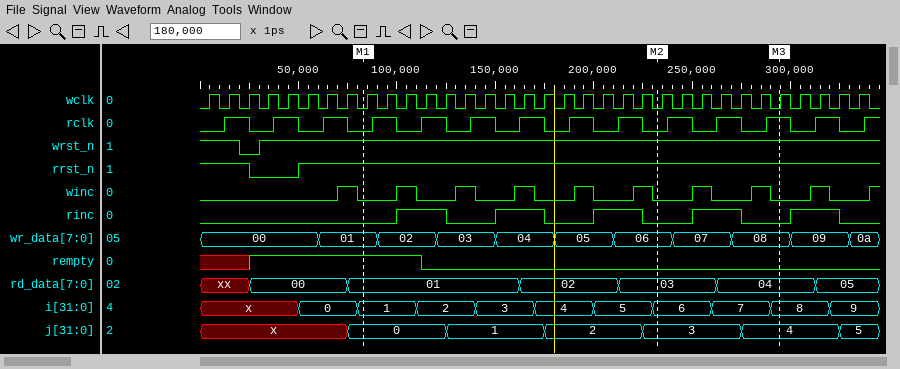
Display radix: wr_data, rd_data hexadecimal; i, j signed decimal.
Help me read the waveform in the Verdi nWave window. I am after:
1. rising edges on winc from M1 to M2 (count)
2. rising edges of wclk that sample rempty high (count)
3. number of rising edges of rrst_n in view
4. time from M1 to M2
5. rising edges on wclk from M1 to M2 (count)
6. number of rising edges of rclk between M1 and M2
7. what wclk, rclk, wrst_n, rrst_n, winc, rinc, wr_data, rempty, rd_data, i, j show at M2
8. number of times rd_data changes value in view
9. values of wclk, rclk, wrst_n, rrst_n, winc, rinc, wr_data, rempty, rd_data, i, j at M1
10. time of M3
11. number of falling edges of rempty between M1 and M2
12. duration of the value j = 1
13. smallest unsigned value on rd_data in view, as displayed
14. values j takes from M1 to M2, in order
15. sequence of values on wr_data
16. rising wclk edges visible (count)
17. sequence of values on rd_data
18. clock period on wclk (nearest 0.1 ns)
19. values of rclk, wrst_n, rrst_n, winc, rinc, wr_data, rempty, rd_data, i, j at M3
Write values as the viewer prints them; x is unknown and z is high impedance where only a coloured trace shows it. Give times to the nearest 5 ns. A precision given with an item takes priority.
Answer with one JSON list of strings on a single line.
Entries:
["5", "8", "1", "150 ns", "15", "6", "wclk=0, rclk=0, wrst_n=1, rrst_n=1, winc=0, rinc=0, wr_data=06, rempty=0, rd_data=03, i=6, j=3", "6", "wclk=0, rclk=0, wrst_n=1, rrst_n=1, winc=0, rinc=0, wr_data=01, rempty=1, rd_data=01, i=1, j=0", "295 ns", "1", "50 ns", "00", "0, 1, 2, 3", "00, 01, 02, 03, 04, 05, 06, 07, 08, 09, 0a", "34", "xx, 00, 01, 02, 03, 04, 05", "10 ns", "rclk=1, wrst_n=1, rrst_n=1, winc=0, rinc=0, wr_data=08, rempty=0, rd_data=04, i=8, j=4"]
